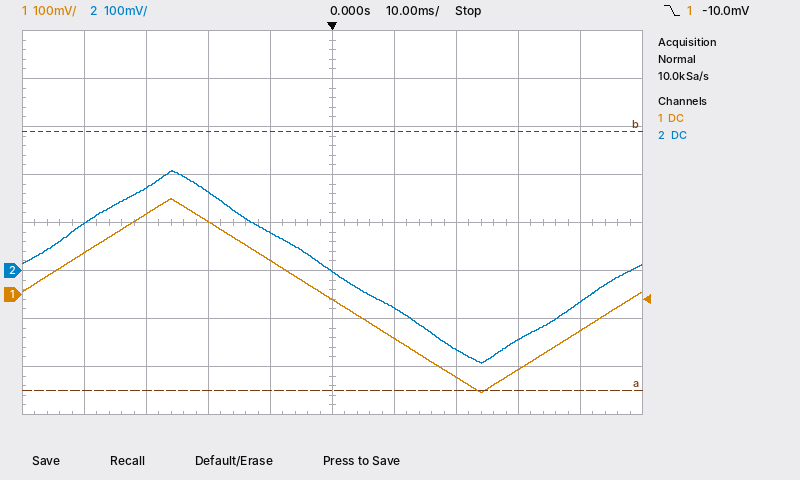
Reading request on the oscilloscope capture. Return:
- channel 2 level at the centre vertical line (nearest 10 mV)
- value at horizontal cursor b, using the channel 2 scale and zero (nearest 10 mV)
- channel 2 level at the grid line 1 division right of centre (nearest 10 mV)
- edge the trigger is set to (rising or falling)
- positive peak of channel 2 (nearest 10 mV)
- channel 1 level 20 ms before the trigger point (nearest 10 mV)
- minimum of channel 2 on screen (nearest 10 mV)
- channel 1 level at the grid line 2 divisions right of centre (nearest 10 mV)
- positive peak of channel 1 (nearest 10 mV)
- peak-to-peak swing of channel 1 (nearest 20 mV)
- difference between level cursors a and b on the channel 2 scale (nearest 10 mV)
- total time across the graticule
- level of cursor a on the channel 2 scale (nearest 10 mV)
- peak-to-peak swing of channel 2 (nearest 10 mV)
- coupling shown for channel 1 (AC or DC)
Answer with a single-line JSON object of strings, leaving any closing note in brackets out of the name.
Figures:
{"channel 2 level at the centre vertical line": "0 mV", "value at horizontal cursor b, using the channel 2 scale and zero": "290 mV", "channel 2 level at the grid line 1 division right of centre": "-80 mV", "edge the trigger is set to": "falling", "positive peak of channel 2": "210 mV", "channel 1 level 20 ms before the trigger point": "150 mV", "minimum of channel 2 on screen": "-190 mV", "channel 1 level at the grid line 2 divisions right of centre": "-170 mV", "positive peak of channel 1": "200 mV", "peak-to-peak swing of channel 1": "400 mV", "difference between level cursors a and b on the channel 2 scale": "540 mV", "total time across the graticule": "100 ms", "level of cursor a on the channel 2 scale": "-250 mV", "peak-to-peak swing of channel 2": "400 mV", "coupling shown for channel 1": "DC"}
